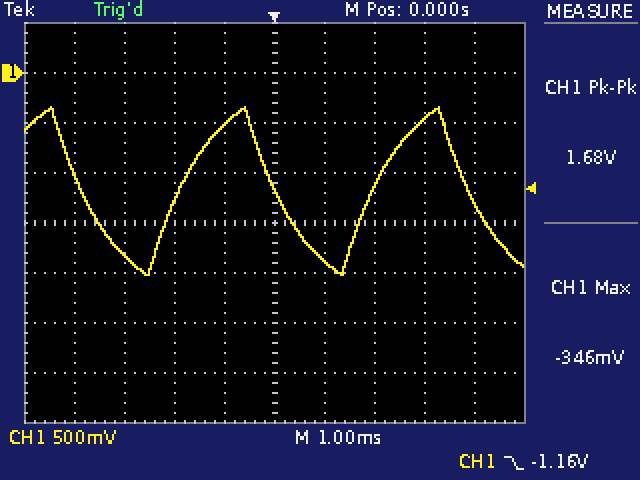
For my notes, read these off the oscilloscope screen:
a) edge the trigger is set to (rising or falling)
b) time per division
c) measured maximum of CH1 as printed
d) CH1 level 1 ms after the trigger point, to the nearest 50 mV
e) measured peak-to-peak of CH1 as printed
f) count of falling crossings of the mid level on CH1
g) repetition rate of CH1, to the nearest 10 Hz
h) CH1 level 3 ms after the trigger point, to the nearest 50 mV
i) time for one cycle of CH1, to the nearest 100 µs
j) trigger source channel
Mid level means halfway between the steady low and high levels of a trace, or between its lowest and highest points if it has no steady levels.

falling
1 ms
-346 mV
-1.90 V
1.68 V
3
260 Hz
-450 mV
3.9 ms
CH1
